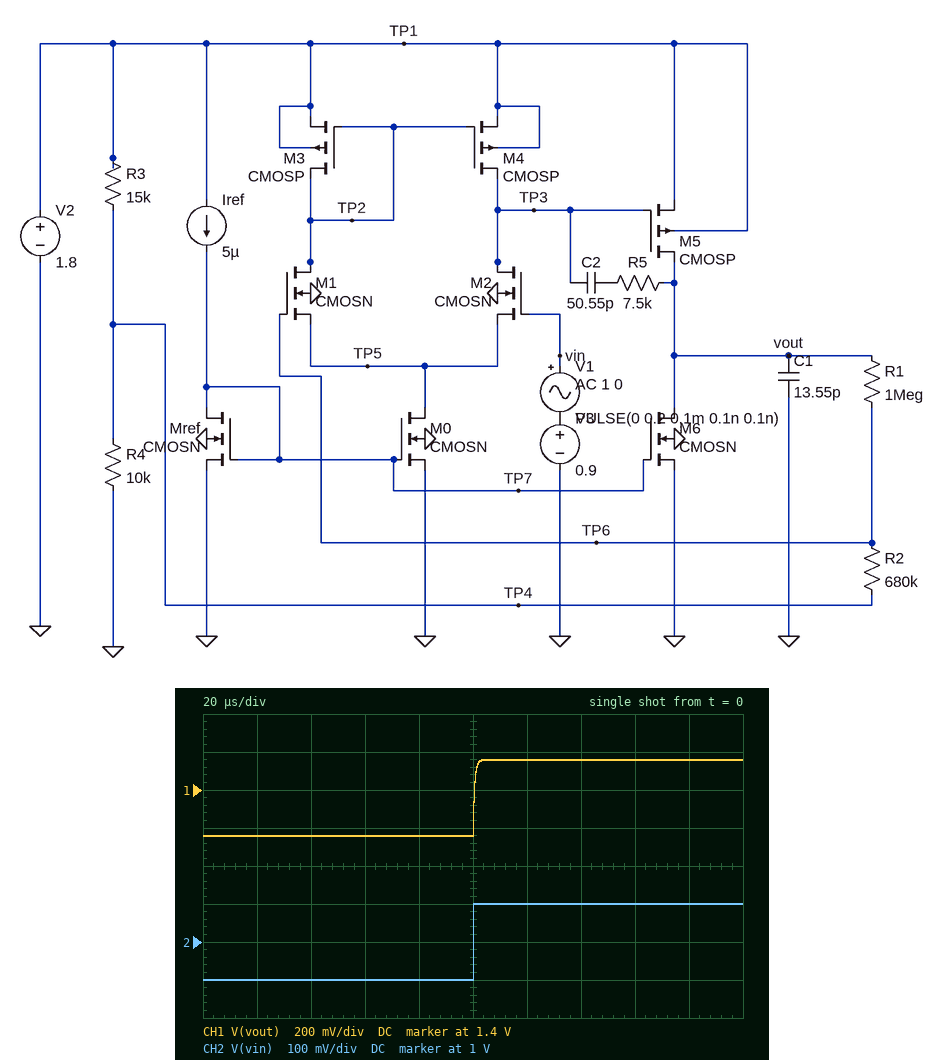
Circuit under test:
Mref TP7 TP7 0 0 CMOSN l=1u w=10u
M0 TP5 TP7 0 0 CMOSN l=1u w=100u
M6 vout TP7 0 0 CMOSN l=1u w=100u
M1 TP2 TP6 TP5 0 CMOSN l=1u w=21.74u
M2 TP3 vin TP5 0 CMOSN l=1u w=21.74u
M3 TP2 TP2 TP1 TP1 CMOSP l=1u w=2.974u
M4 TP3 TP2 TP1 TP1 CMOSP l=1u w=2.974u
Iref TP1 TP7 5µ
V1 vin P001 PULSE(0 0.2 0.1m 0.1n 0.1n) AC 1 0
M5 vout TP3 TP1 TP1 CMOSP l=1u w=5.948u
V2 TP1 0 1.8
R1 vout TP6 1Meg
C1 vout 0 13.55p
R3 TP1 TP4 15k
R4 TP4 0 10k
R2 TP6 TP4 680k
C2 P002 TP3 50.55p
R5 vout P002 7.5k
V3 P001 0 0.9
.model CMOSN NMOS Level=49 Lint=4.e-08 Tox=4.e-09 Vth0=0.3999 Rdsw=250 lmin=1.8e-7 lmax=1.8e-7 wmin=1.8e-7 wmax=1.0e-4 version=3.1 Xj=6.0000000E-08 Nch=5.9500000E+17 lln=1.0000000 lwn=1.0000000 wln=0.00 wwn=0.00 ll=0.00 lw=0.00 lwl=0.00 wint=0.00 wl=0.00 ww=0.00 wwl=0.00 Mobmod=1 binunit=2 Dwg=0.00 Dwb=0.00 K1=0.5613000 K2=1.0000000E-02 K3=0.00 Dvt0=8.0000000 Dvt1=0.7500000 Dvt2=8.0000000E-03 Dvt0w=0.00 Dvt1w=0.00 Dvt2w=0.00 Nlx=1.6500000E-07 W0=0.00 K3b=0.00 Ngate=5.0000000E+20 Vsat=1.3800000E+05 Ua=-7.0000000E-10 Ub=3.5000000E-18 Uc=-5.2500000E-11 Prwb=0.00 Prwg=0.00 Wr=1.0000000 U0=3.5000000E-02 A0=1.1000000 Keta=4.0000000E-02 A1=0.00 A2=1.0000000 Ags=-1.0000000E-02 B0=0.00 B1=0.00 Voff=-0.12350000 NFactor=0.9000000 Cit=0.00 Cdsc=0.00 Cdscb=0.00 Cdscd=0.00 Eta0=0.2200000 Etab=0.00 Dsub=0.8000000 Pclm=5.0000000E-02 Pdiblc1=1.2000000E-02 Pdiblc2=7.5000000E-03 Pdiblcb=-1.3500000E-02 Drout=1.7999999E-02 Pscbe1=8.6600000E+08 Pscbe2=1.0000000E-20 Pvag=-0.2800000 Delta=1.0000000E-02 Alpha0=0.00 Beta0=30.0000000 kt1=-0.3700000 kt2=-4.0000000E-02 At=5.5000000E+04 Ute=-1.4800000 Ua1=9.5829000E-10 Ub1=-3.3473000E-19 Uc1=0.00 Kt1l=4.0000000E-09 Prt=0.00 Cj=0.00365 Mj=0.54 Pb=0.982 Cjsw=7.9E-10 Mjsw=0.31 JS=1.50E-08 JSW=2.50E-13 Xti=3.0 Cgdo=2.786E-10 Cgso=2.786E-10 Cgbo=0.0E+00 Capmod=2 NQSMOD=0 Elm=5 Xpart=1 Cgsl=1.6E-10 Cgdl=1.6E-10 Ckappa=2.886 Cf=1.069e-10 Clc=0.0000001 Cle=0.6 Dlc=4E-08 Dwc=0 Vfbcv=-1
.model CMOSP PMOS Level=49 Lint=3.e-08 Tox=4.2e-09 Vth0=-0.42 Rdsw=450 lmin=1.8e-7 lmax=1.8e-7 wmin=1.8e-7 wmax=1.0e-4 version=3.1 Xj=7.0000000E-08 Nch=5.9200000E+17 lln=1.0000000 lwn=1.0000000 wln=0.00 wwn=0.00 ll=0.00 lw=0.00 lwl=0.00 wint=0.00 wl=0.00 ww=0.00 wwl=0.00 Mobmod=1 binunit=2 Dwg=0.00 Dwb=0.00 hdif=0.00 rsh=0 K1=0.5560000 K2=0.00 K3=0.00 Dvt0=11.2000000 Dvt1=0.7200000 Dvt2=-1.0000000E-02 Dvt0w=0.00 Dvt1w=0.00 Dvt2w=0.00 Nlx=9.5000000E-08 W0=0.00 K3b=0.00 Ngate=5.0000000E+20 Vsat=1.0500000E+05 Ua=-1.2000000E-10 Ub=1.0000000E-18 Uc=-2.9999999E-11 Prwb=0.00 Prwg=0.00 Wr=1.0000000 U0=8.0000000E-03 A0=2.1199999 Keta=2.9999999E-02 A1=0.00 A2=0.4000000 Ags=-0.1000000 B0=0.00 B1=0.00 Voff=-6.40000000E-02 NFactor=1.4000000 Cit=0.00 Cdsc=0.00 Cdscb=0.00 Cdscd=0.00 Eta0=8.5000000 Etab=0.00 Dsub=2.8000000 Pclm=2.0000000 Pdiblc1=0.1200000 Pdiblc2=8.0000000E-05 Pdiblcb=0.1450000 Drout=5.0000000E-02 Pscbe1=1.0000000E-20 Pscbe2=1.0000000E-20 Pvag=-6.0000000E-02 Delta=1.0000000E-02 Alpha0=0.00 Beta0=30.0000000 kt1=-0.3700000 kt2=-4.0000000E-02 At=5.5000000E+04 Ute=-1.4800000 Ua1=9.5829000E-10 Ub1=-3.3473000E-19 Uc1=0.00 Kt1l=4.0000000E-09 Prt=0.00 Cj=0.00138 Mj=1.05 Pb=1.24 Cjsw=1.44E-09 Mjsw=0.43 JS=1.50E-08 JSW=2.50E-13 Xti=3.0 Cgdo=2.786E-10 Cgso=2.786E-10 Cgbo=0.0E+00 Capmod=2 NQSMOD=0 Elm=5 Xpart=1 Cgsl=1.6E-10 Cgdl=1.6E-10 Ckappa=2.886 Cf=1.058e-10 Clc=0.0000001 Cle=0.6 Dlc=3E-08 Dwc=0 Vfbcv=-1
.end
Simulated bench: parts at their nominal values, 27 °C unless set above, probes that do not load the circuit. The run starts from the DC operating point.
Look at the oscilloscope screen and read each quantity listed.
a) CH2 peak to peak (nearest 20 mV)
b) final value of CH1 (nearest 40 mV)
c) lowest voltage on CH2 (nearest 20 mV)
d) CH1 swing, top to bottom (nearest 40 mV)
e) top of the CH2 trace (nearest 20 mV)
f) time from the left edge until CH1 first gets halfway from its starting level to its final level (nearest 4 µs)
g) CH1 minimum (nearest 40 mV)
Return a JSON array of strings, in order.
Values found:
["200 mV", "1.56 V", "900 mV", "400 mV", "1.10 V", "100 µs", "1.16 V"]
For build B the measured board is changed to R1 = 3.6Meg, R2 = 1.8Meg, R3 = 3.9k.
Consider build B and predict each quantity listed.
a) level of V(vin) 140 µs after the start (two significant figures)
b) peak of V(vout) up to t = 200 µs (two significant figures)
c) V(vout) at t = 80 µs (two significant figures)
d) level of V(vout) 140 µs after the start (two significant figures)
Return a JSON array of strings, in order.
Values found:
["1.1 V", "720 mV", "110 mV", "710 mV"]
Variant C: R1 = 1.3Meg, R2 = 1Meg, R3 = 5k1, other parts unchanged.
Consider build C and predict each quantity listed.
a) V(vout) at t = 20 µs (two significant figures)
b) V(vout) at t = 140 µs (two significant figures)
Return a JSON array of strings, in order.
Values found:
["520 mV", "980 mV"]
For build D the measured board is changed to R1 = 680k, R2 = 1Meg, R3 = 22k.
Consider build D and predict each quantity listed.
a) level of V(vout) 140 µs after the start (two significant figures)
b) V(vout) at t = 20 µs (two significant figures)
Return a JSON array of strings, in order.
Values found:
["1.5 V", "1.1 V"]
